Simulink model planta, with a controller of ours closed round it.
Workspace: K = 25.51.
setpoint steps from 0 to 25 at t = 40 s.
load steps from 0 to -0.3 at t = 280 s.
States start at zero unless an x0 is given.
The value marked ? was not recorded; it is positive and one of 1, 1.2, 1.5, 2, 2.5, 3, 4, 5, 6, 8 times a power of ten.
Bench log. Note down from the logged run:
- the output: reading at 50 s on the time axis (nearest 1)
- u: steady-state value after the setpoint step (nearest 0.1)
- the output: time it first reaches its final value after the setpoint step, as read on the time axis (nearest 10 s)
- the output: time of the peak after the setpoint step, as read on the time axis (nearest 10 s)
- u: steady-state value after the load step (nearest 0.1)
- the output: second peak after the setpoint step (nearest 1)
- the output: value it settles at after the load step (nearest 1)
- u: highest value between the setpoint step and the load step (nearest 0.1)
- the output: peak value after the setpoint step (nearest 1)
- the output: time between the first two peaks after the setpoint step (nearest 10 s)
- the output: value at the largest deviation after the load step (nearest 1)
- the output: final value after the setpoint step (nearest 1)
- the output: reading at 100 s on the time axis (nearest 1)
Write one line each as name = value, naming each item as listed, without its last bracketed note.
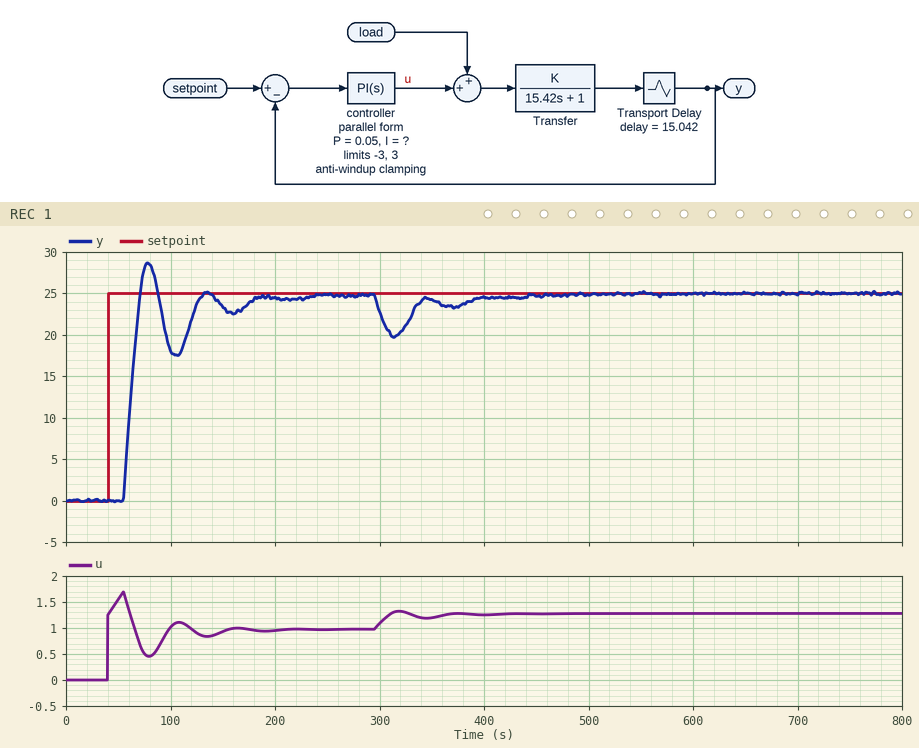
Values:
the output: reading at 50 s on the time axis = 0
u: steady-state value after the setpoint step = 1.0
the output: time it first reaches its final value after the setpoint step, as read on the time axis = 70 s
the output: time of the peak after the setpoint step, as read on the time axis = 80 s
u: steady-state value after the load step = 1.3
the output: second peak after the setpoint step = 25
the output: value it settles at after the load step = 25
u: highest value between the setpoint step and the load step = 1.7
the output: peak value after the setpoint step = 29
the output: time between the first two peaks after the setpoint step = 60 s
the output: value at the largest deviation after the load step = 20
the output: final value after the setpoint step = 25
the output: reading at 100 s on the time axis = 18
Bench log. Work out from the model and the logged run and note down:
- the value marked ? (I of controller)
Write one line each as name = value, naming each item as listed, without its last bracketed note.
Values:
the value marked ? = 0.0012
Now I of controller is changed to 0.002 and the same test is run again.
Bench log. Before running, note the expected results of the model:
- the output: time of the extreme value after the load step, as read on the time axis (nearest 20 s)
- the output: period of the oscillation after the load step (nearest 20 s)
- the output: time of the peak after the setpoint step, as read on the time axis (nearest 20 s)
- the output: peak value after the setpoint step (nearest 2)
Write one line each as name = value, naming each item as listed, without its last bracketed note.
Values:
the output: time of the extreme value after the load step, as read on the time axis = 320 s
the output: period of the oscillation after the load step = 60 s
the output: time of the peak after the setpoint step, as read on the time axis = 80 s
the output: peak value after the setpoint step = 34
